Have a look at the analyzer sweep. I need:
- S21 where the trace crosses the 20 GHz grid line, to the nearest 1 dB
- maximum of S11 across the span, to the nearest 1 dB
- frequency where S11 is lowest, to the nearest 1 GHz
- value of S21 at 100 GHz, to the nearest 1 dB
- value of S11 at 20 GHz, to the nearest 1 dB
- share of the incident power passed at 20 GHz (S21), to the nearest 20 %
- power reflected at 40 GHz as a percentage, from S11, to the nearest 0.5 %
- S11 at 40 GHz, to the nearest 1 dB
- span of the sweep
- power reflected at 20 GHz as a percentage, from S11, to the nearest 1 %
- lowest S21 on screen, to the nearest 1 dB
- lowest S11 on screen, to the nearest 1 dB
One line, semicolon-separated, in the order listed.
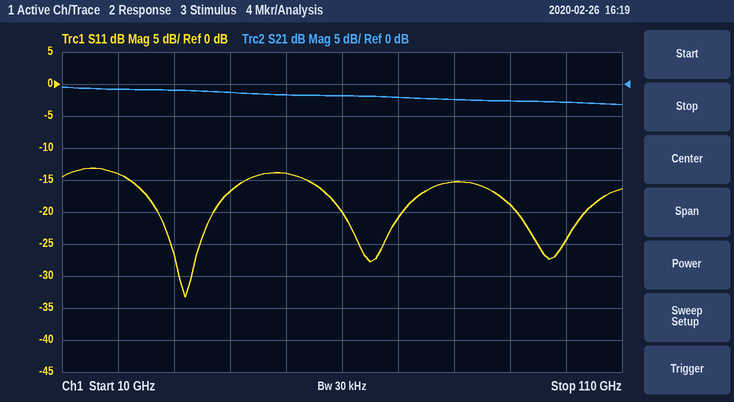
-1 dB; -13 dB; 32 GHz; -3 dB; -14 dB; 80 %; 2.0 %; -17 dB; 100 GHz; 4 %; -3 dB; -33 dB
